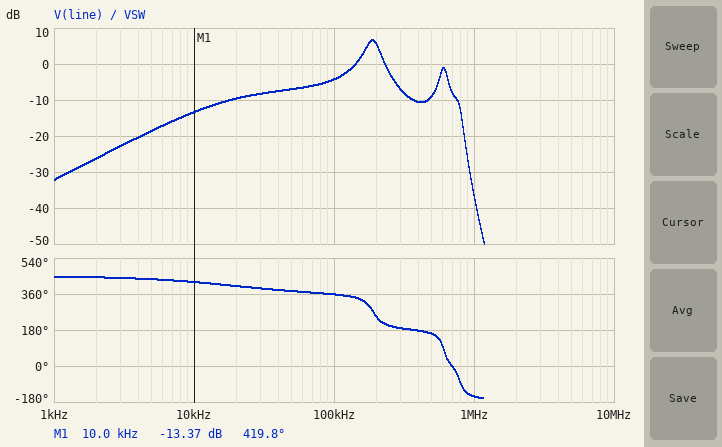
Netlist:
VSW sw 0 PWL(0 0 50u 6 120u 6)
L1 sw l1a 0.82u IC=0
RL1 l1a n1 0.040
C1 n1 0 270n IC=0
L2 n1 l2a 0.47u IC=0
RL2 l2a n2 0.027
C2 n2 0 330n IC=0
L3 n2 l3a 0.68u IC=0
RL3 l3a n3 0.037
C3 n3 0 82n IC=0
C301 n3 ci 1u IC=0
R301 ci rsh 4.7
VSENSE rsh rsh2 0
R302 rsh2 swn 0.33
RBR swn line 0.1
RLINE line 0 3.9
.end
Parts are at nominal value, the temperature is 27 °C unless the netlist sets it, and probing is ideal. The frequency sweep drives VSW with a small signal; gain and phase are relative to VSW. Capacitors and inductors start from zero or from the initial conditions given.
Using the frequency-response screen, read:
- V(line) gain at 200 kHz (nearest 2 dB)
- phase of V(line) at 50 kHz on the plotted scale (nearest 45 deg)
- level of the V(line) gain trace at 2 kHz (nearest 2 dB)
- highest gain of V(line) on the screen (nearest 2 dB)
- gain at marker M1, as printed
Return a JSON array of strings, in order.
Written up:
["6 dB", "360 deg", "-26 dB", "6 dB", "-13.37 dB"]
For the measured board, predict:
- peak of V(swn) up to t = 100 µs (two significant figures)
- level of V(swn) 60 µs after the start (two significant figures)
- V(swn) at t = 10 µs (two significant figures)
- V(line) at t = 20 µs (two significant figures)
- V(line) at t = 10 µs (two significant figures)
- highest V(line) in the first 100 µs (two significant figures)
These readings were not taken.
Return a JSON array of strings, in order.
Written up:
["480 mV", "150 mV", "330 mV", "420 mV", "320 mV", "470 mV"]
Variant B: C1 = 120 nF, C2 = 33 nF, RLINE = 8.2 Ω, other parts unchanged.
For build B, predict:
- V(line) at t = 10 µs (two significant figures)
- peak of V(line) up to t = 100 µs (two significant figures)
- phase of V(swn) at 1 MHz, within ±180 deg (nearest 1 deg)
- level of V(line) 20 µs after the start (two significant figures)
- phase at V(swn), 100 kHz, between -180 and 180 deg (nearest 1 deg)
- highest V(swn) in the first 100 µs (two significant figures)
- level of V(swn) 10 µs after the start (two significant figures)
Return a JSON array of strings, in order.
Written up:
["510 mV", "960 mV", "14 deg", "760 mV", "0 deg", "970 mV", "520 mV"]
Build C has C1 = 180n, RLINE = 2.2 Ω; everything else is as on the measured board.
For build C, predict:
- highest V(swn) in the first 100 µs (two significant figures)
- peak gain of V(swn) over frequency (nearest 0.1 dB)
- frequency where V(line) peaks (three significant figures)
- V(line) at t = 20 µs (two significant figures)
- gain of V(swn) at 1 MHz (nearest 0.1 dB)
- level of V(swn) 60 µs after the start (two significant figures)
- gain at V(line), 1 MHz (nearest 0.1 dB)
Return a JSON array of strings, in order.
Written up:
["280 mV", "1.8 dB", "196 kHz", "250 mV", "-33.1 dB", "68 mV", "-33.5 dB"]
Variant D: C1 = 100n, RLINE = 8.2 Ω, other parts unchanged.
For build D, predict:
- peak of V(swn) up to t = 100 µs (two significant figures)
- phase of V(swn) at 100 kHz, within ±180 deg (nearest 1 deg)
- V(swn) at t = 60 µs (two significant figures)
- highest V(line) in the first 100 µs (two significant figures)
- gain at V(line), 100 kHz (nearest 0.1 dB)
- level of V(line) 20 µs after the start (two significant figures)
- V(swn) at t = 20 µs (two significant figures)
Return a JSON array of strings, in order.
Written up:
["970 mV", "-1 deg", "470 mV", "960 mV", "-1.7 dB", "760 mV", "770 mV"]
